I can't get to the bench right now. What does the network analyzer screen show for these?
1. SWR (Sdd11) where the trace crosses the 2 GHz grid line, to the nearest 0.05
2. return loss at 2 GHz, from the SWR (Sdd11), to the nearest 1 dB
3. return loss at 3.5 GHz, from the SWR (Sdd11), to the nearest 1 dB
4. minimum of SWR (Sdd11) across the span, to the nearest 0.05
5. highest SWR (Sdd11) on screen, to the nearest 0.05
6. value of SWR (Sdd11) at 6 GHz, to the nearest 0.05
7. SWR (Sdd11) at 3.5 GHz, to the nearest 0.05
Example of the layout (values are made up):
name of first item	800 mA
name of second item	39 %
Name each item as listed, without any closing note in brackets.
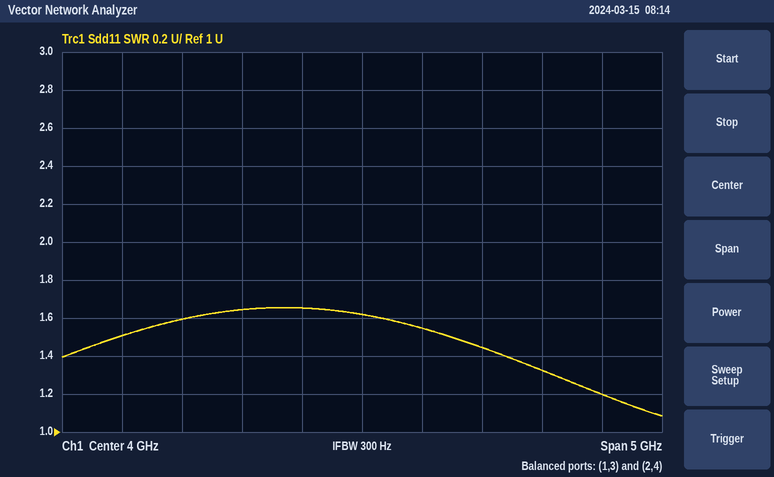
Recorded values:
SWR (Sdd11) where the trace crosses the 2 GHz grid line, to the nearest 0.05	1.50
return loss at 2 GHz, from the SWR (Sdd11), to the nearest 1 dB	14 dB
return loss at 3.5 GHz, from the SWR (Sdd11), to the nearest 1 dB	12 dB
minimum of SWR (Sdd11) across the span, to the nearest 0.05	1.10
highest SWR (Sdd11) on screen, to the nearest 0.05	1.65
value of SWR (Sdd11) at 6 GHz, to the nearest 0.05	1.20
SWR (Sdd11) at 3.5 GHz, to the nearest 0.05	1.65
